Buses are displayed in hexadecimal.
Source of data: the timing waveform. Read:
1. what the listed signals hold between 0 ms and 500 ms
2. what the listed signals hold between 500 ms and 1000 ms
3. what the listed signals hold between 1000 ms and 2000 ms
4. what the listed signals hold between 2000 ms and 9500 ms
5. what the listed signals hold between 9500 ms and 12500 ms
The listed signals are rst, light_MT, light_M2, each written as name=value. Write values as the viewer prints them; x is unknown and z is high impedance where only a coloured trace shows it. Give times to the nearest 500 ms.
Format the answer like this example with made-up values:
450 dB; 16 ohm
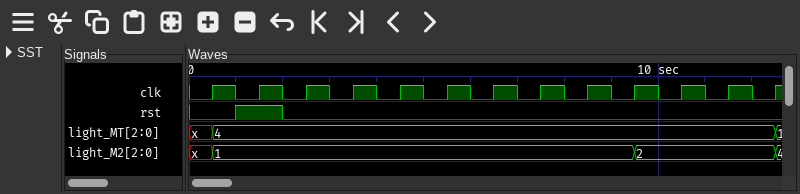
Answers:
rst=0, light_MT=x, light_M2=x; rst=0, light_MT=4, light_M2=1; rst=1, light_MT=4, light_M2=1; rst=0, light_MT=4, light_M2=1; rst=0, light_MT=4, light_M2=2
